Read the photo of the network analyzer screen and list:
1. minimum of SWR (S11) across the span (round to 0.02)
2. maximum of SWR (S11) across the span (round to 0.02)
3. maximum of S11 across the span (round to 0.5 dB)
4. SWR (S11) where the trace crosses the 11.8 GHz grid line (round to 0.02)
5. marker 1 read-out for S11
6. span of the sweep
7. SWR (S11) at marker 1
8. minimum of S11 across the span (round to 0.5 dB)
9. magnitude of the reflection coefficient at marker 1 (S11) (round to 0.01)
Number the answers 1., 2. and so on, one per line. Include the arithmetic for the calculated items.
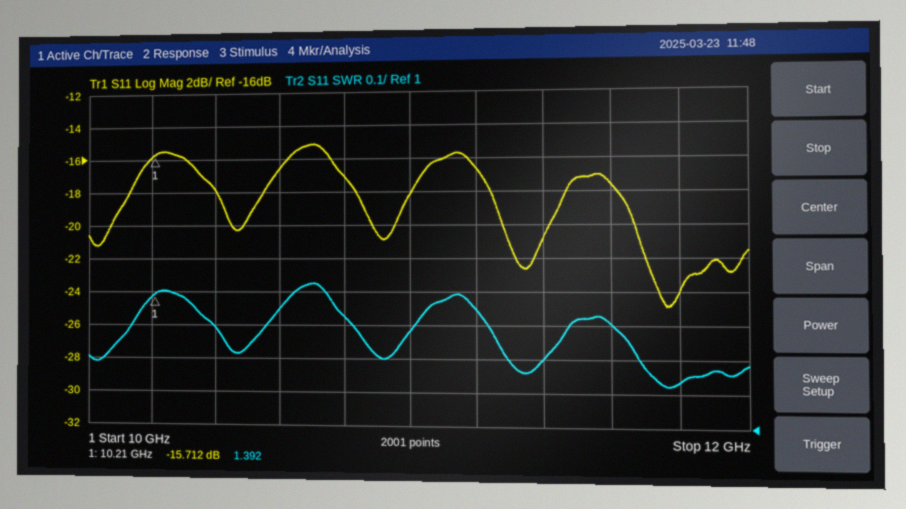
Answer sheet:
1. 1.12
2. 1.42
3. -15.0 dB
4. 1.14
5. -15.712 dB
6. 2 GHz
7. 1.392
8. -25.0 dB
9. 10^(-15.712/20) ≈ 0.16
